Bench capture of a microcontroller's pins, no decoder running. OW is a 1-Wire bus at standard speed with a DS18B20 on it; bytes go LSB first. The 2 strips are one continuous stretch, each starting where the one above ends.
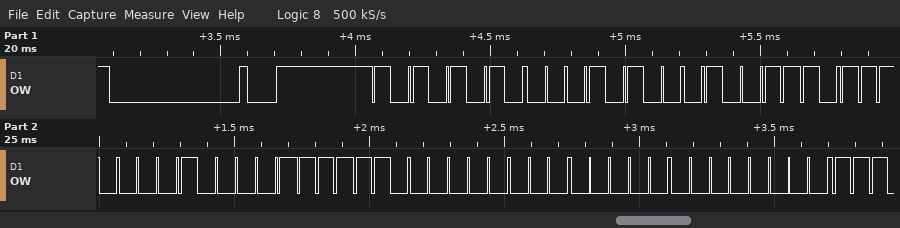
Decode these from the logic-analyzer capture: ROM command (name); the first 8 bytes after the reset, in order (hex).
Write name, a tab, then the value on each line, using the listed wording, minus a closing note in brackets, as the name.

ROM command	Match ROM
the first 8 bytes after the reset, in order	55 28 72 87 F0 03 00 00
